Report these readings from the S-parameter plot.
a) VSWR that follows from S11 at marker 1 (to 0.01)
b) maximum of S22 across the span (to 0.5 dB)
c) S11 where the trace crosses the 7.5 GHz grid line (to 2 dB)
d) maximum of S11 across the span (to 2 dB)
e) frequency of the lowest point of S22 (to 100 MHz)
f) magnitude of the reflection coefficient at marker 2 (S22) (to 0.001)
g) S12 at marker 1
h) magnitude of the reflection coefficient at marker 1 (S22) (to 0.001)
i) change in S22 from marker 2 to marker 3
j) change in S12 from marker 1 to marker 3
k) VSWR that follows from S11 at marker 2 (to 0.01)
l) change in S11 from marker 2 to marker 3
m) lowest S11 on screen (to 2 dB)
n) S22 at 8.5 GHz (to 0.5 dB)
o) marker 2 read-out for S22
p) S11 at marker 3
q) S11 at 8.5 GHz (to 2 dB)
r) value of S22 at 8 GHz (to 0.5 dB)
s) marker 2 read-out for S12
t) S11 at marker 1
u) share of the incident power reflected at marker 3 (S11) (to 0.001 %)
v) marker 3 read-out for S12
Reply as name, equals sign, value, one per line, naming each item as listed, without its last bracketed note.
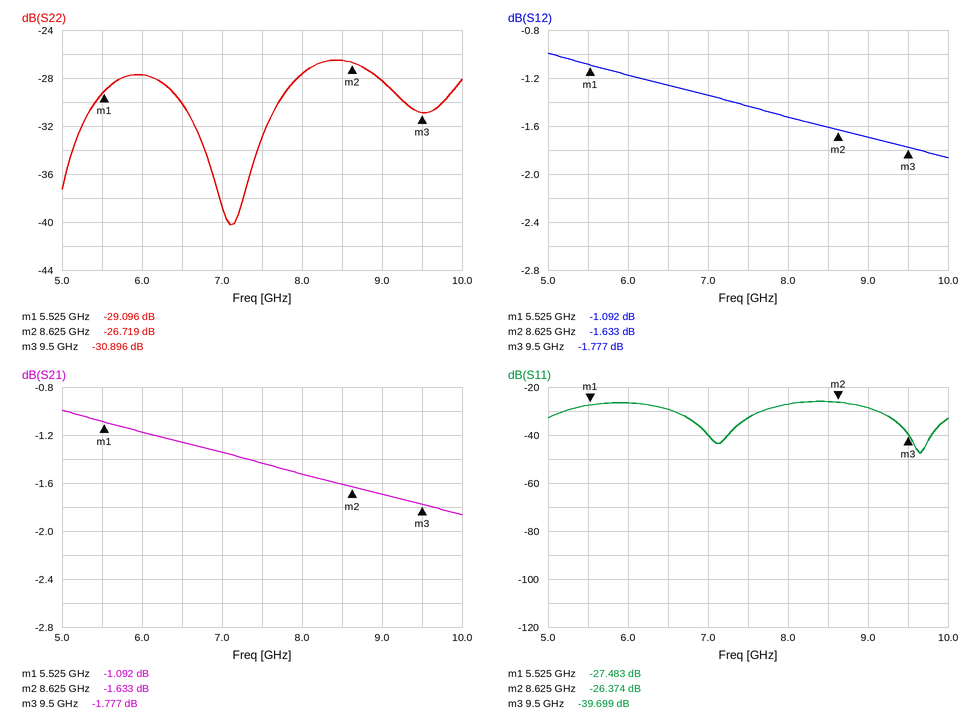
VSWR that follows from S11 at marker 1 = 1.09
maximum of S22 across the span = -26.5 dB
S11 where the trace crosses the 7.5 GHz grid line = -32 dB
maximum of S11 across the span = -26 dB
frequency of the lowest point of S22 = 7.1 GHz
magnitude of the reflection coefficient at marker 2 (S22) = 0.046
S12 at marker 1 = -1.092 dB
magnitude of the reflection coefficient at marker 1 (S22) = 0.035
change in S22 from marker 2 to marker 3 = -4.177 dB
change in S12 from marker 1 to marker 3 = -0.685 dB
VSWR that follows from S11 at marker 2 = 1.10
change in S11 from marker 2 to marker 3 = -13.325 dB
lowest S11 on screen = -48 dB
S22 at 8.5 GHz = -26.5 dB
marker 2 read-out for S22 = -26.719 dB
S11 at marker 3 = -39.699 dB
S11 at 8.5 GHz = -26 dB
value of S22 at 8 GHz = -27.5 dB
marker 2 read-out for S12 = -1.633 dB
S11 at marker 1 = -27.483 dB
share of the incident power reflected at marker 3 (S11) = 0.011 %
marker 3 read-out for S12 = -1.777 dB
